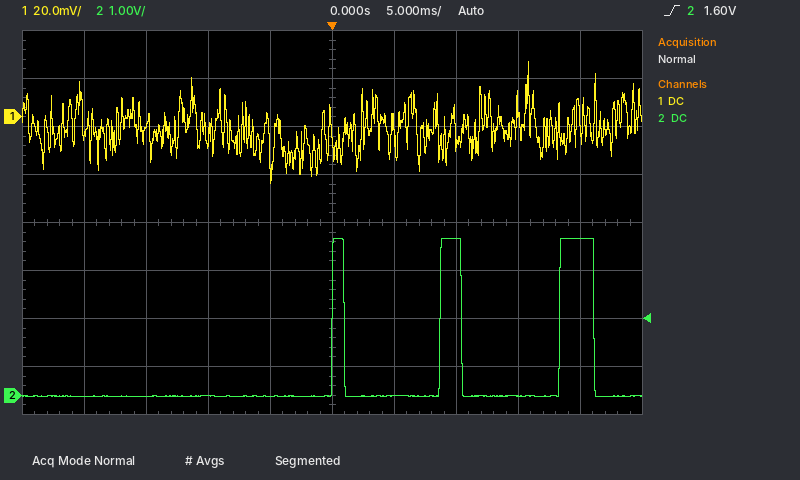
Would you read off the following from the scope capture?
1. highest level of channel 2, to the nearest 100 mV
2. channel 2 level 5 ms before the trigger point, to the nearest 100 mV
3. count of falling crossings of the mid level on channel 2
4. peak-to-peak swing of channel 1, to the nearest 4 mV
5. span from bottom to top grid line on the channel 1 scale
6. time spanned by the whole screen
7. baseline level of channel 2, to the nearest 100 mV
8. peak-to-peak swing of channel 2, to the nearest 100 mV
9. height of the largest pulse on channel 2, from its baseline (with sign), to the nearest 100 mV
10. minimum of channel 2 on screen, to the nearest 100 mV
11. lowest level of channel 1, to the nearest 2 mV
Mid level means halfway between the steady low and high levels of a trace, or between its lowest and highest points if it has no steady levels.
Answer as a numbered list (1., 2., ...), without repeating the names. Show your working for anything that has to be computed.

1. 3.3 V
2. 0.0 V
3. 3
4. 52 mV
5. 160 mV
6. 50 ms
7. 0.0 V
8. 3.3 V − (0.0 V) = 3.3 V
9. 3.3 V − (0.0 V) = +3.3 V
10. 0.0 V
11. -28 mV
